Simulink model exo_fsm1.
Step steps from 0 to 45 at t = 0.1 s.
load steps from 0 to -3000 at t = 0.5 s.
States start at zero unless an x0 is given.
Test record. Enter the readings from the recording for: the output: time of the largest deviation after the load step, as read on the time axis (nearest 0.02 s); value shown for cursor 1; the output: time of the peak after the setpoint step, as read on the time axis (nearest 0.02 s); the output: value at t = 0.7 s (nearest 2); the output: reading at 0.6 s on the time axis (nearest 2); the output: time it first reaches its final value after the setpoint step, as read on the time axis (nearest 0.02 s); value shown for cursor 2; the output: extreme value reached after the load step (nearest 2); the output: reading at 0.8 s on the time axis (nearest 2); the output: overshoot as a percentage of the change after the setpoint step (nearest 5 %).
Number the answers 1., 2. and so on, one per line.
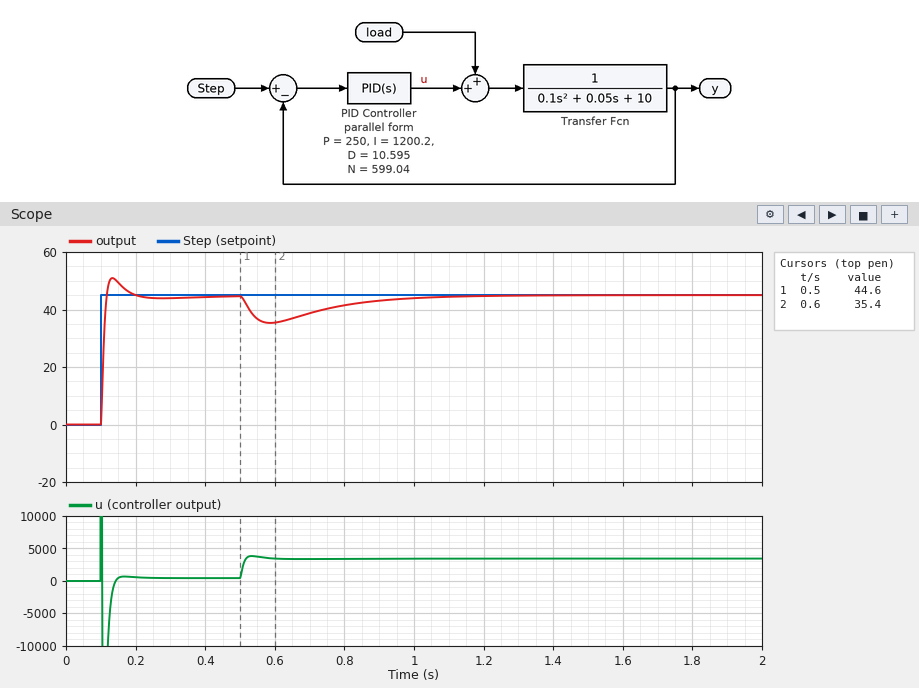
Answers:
1. 0.58 s
2. 44.6
3. 0.14 s
4. 38
5. 36
6. 0.12 s
7. 35.4
8. 36
9. 42
10. 15 %
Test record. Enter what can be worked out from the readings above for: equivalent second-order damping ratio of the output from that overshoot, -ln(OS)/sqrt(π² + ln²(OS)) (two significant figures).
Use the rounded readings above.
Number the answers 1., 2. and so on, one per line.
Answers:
1. 0.52
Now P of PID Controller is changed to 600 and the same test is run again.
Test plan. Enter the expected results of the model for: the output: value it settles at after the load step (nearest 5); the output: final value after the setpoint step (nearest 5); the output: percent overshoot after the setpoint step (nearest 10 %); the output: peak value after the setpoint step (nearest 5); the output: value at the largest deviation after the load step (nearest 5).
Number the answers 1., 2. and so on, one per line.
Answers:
1. 45
2. 45
3. 20 %
4. 55
5. 40
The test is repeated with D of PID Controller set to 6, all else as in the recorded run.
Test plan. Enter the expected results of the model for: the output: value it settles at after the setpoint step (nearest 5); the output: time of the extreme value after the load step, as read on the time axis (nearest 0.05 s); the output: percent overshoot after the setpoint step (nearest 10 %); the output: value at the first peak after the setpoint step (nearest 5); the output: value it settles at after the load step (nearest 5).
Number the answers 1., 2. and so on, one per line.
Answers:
1. 45
2. 0.55 s
3. 30 %
4. 55
5. 45
